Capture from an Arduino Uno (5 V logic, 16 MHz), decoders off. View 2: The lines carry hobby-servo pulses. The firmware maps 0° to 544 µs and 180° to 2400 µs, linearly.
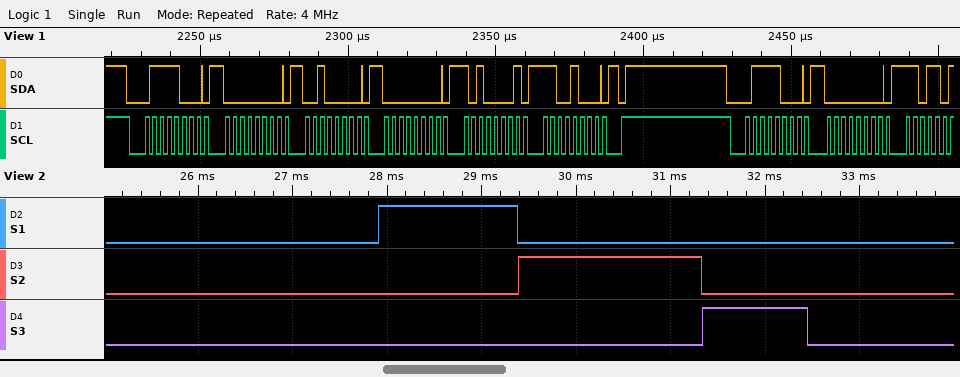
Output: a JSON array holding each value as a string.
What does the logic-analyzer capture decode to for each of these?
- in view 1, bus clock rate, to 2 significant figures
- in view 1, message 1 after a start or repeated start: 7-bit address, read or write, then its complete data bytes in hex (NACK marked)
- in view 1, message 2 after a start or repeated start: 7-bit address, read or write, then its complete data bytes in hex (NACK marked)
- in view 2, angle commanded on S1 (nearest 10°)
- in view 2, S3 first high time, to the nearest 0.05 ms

["400 kHz", "0x3C write: 00 20 00 A1 C8", "0x3C write: 00", "90°", "1.10 ms"]
